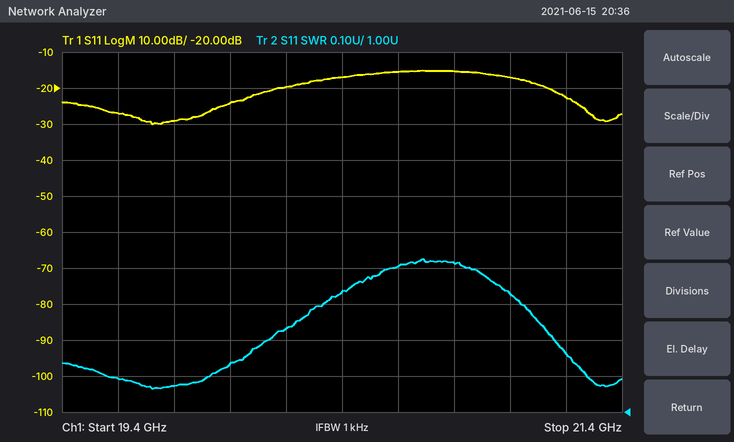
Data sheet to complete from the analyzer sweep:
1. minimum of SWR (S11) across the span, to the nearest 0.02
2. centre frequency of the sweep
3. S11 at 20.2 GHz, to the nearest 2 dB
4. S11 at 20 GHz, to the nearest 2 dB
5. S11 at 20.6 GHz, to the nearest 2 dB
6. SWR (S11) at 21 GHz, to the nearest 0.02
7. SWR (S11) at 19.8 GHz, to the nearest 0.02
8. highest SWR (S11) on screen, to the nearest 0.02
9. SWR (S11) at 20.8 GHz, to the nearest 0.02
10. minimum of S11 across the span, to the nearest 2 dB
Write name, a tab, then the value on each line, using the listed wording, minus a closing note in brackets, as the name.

minimum of SWR (S11) across the span, to the nearest 0.02	1.06
centre frequency of the sweep	20.4 GHz
S11 at 20.2 GHz, to the nearest 2 dB	-20 dB
S11 at 20 GHz, to the nearest 2 dB	-24 dB
S11 at 20.6 GHz, to the nearest 2 dB	-16 dB
SWR (S11) at 21 GHz, to the nearest 0.02	1.32
SWR (S11) at 19.8 GHz, to the nearest 0.02	1.08
highest SWR (S11) on screen, to the nearest 0.02	1.42
SWR (S11) at 20.8 GHz, to the nearest 0.02	1.42
minimum of S11 across the span, to the nearest 2 dB	-30 dB
